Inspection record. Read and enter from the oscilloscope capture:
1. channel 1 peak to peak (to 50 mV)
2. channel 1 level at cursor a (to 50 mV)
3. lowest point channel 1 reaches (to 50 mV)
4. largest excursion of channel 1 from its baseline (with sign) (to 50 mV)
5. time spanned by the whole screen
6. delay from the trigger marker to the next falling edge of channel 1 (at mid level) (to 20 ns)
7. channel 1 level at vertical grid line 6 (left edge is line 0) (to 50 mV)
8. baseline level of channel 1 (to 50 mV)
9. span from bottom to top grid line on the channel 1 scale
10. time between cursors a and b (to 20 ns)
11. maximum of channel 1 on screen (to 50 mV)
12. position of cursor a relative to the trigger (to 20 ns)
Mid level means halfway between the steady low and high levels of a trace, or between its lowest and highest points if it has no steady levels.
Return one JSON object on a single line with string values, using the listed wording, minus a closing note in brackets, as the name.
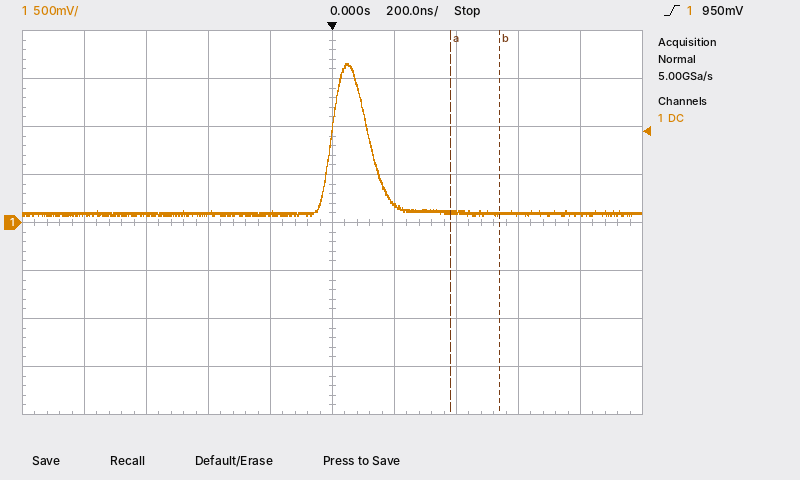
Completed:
{"channel 1 peak to peak": "1.60 V", "channel 1 level at cursor a": "100 mV", "lowest point channel 1 reaches": "50 mV", "largest excursion of channel 1 from its baseline (with sign)": "+1.55 V", "time spanned by the whole screen": "2 µs", "delay from the trigger marker to the next falling edge of channel 1 (at mid level)": "120 ns", "channel 1 level at vertical grid line 6 (left edge is line 0)": "200 mV", "baseline level of channel 1": "100 mV", "span from bottom to top grid line on the channel 1 scale": "4 V", "time between cursors a and b": "160 ns", "maximum of channel 1 on screen": "1.65 V", "position of cursor a relative to the trigger": "+380 ns"}
